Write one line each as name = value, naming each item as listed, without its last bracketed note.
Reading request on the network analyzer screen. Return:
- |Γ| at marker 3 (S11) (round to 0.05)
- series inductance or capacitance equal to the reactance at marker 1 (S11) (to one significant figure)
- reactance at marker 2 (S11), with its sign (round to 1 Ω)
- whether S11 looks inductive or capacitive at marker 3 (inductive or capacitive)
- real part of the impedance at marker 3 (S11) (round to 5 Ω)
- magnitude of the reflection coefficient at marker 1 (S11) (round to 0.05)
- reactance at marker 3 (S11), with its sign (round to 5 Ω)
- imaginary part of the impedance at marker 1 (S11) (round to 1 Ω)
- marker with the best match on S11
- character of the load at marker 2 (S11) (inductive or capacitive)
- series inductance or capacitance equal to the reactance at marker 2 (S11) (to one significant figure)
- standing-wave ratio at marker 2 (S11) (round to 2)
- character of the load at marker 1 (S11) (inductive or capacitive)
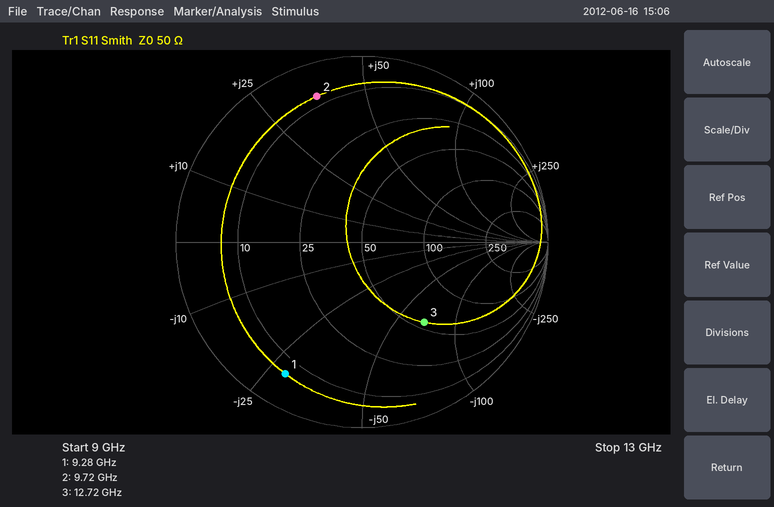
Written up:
|Γ| at marker 3 (S11) = 0.55
series inductance or capacitance equal to the reactance at marker 1 (S11) = 600 fF
reactance at marker 2 (S11), with its sign = +36 Ω
whether S11 looks inductive or capacitive at marker 3 = capacitive
real part of the impedance at marker 3 (S11) = 55 Ω
magnitude of the reflection coefficient at marker 1 (S11) = 0.80
reactance at marker 3 (S11), with its sign = -70 Ω
imaginary part of the impedance at marker 1 (S11) = -28 Ω
marker with the best match on S11 = marker 3
character of the load at marker 2 (S11) = inductive
series inductance or capacitance equal to the reactance at marker 2 (S11) = 600 pH
standing-wave ratio at marker 2 (S11) = 10
character of the load at marker 1 (S11) = capacitive
